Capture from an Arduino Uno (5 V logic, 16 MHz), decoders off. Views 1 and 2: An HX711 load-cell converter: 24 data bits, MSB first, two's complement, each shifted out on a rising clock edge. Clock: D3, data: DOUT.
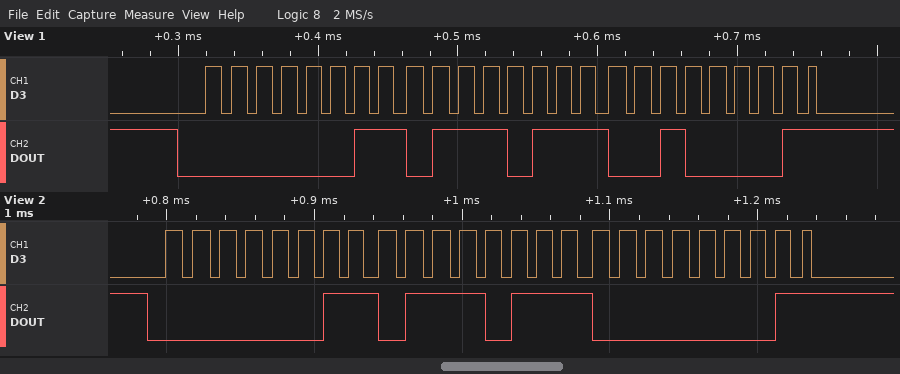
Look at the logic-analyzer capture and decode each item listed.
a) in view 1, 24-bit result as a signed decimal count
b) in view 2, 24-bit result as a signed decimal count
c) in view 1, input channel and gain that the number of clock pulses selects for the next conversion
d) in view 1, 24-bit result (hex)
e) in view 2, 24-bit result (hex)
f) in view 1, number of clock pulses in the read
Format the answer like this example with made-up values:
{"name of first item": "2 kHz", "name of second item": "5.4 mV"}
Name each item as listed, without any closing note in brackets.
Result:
{"in view 1, 24-bit result as a signed decimal count": "227105", "in view 2, 24-bit result as a signed decimal count": "227073", "in view 1, input channel and gain that the number of clock pulses selects for the next conversion": "channel A, gain 128", "in view 1, 24-bit result": "0x037721", "in view 2, 24-bit result": "0x037701", "in view 1, number of clock pulses in the read": "25"}
